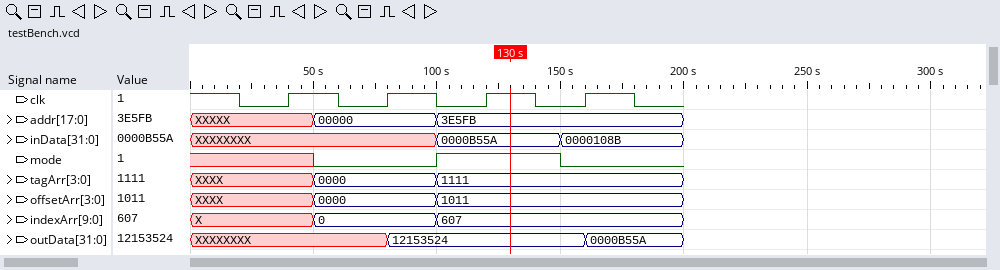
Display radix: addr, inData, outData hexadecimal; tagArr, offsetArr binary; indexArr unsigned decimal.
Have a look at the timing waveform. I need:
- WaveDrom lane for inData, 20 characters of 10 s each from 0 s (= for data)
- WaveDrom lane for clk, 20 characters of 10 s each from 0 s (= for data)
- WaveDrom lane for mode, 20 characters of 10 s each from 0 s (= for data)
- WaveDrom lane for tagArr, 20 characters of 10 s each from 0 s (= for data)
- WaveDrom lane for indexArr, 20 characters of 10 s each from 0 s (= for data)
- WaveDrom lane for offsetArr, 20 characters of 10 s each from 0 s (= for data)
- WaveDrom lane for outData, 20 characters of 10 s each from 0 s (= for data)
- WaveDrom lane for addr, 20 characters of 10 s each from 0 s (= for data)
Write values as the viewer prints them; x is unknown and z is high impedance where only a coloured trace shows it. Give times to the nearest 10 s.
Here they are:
{name: 'inData', wave: 'x.........=....=....', data: '0000B55A 0000108B'}
{name: 'clk', wave: '1.0.1.0.1.0.1.0.1.0.'}
{name: 'mode', wave: 'x....0....1....0....'}
{name: 'tagArr', wave: 'x....=....=.........', data: '0000 1111'}
{name: 'indexArr', wave: 'x....=....=.........', data: '0 607'}
{name: 'offsetArr', wave: 'x....=....=.........', data: '0000 1011'}
{name: 'outData', wave: 'x.......=.......=...', data: '12153524 0000B55A'}
{name: 'addr', wave: 'x....=....=.........', data: '00000 3E5FB'}
